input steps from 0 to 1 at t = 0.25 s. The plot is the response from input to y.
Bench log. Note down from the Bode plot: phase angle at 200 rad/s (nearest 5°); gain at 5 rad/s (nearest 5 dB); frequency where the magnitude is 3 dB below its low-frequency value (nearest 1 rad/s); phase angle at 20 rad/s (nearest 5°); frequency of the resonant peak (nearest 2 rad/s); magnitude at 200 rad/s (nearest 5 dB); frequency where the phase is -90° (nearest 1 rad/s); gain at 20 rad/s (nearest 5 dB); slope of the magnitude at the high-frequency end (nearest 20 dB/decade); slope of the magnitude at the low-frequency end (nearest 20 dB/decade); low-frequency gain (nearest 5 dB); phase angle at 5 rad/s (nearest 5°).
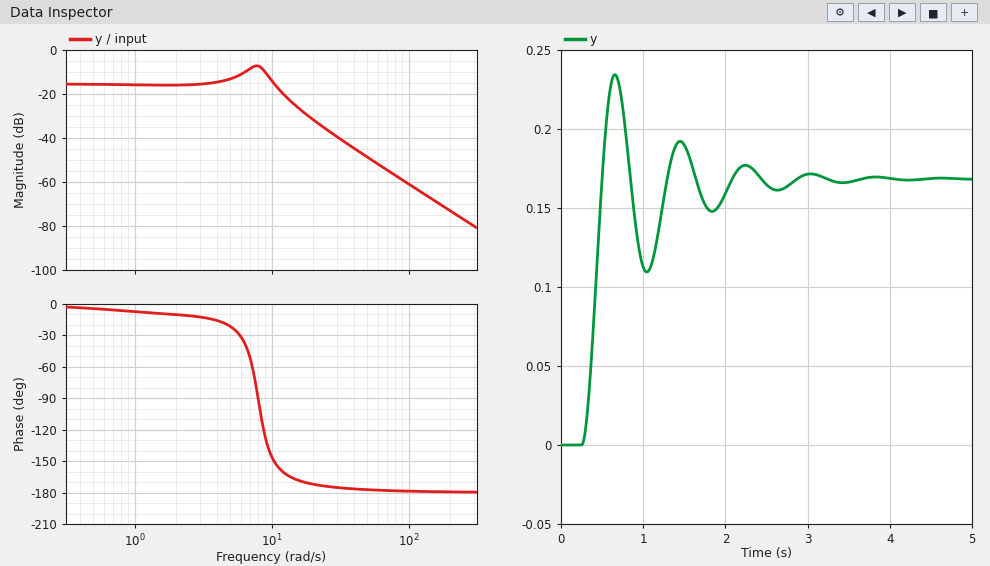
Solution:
-180°
-15 dB
12 rad/s
-170°
8 rad/s
-75 dB
8 rad/s
-30 dB
-40 dB/decade
0 dB/decade
-15 dB
-20°
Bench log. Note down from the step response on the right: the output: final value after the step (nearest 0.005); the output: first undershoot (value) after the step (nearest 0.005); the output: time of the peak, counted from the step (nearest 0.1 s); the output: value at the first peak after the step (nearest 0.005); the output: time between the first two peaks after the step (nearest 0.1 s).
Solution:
0.170
0.110
0.4 s
0.235
0.8 s
